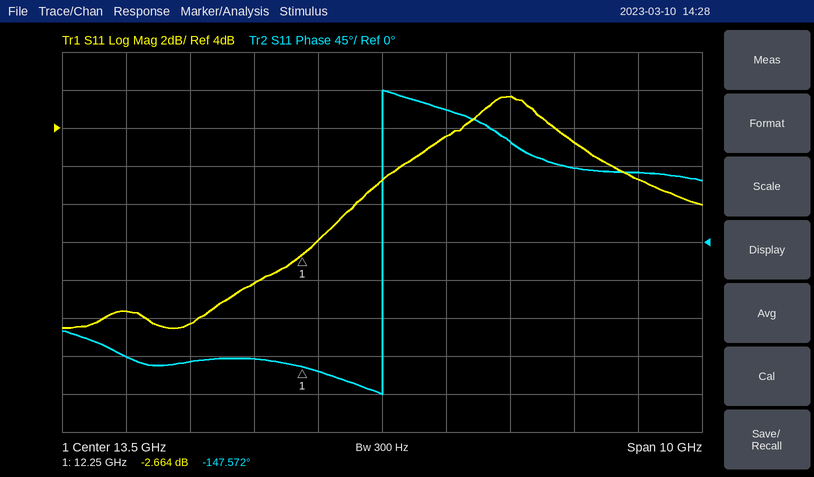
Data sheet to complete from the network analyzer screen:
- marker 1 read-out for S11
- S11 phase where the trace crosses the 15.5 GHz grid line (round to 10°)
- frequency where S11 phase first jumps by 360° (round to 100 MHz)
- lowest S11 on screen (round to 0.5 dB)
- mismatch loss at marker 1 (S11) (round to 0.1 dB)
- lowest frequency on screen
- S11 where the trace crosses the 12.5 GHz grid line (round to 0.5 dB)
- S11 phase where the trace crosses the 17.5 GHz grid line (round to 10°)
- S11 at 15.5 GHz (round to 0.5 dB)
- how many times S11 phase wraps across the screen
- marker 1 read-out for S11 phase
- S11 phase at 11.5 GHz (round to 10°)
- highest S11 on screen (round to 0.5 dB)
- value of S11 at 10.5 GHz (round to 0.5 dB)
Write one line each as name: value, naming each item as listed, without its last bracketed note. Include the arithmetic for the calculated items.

marker 1 read-out for S11: -2.664 dB
S11 phase where the trace crosses the 15.5 GHz grid line: 120°
frequency where S11 phase first jumps by 360°: 13.5 GHz
lowest S11 on screen: -6.5 dB
mismatch loss at marker 1 (S11): −10 log10(1 − 10^(-2.664/10)) ≈ 3.4 dB
lowest frequency on screen: 8.5 GHz
S11 where the trace crosses the 12.5 GHz grid line: -2.0 dB
S11 phase where the trace crosses the 17.5 GHz grid line: 80°
S11 at 15.5 GHz: 5.5 dB
how many times S11 phase wraps across the screen: 1
marker 1 read-out for S11 phase: -147.572°
S11 phase at 11.5 GHz: -140°
highest S11 on screen: 5.5 dB
value of S11 at 10.5 GHz: -6.5 dB
